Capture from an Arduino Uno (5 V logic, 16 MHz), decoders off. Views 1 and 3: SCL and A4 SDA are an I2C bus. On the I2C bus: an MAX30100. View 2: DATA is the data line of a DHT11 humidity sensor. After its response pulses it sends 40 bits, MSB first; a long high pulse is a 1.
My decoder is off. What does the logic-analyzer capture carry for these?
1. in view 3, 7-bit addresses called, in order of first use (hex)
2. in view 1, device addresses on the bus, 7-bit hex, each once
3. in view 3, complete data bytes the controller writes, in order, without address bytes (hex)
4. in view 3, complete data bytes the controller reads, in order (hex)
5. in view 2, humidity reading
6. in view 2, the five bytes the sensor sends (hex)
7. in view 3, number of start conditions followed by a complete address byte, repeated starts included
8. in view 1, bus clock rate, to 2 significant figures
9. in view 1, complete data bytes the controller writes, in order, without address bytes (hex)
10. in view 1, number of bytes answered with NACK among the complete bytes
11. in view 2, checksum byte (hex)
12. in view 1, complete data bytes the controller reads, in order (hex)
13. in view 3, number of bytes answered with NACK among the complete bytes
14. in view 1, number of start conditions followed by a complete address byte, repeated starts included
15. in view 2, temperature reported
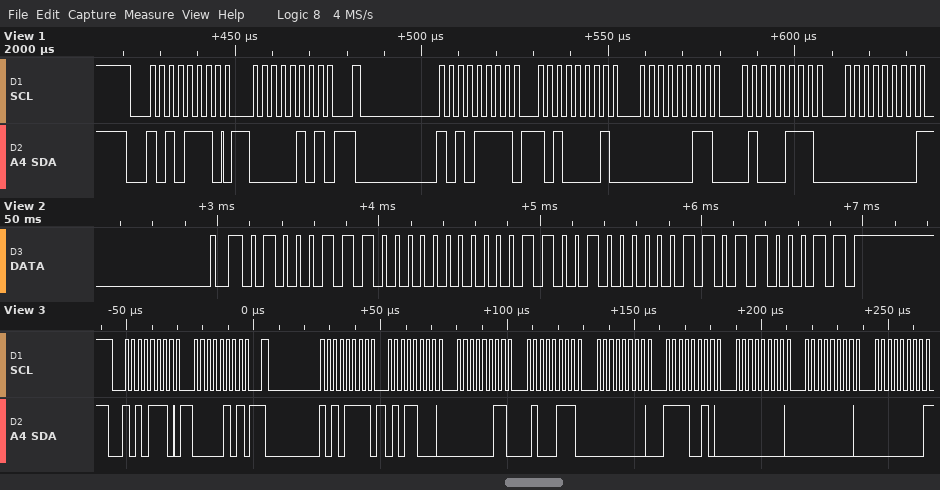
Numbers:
0x57
0x57
05
58 03 47 00 F2 00 00 00
71 %
47 00 19 03 63
2
400 kHz
05
1
0x63
A1 03 47 00
1
2
25.3 °C
